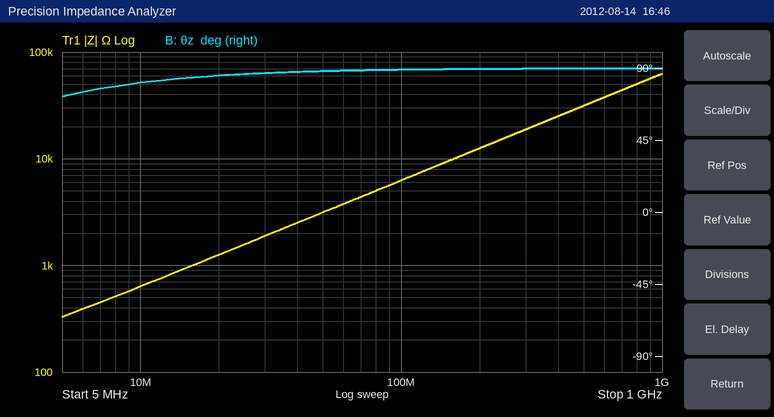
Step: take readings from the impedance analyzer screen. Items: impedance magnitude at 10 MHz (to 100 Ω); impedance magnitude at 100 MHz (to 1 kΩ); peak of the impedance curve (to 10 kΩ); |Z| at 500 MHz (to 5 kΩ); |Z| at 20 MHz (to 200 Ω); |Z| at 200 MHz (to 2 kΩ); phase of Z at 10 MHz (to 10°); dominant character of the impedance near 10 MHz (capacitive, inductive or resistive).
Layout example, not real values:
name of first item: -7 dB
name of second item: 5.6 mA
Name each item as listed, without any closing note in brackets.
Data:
impedance magnitude at 10 MHz: 600 Ω
impedance magnitude at 100 MHz: 6 kΩ
peak of the impedance curve: 60 kΩ
|Z| at 500 MHz: 30 kΩ
|Z| at 20 MHz: 1.2 kΩ
|Z| at 200 MHz: 12 kΩ
phase of Z at 10 MHz: 80°
dominant character of the impedance near 10 MHz: inductive
